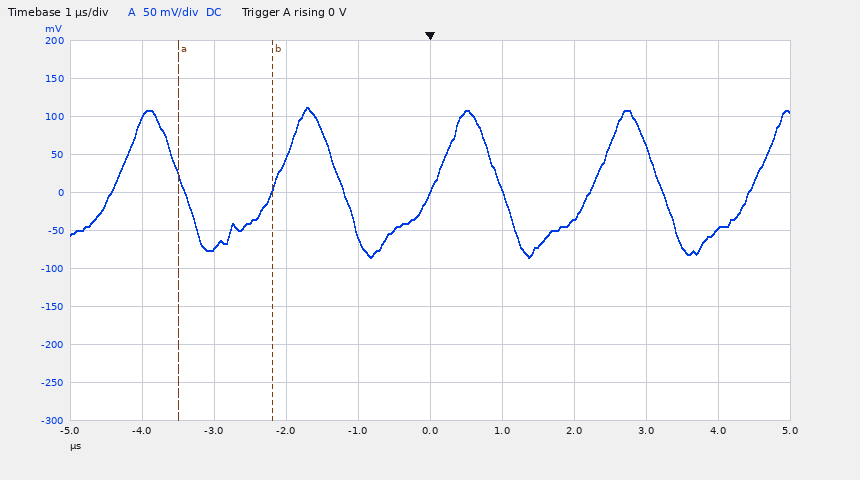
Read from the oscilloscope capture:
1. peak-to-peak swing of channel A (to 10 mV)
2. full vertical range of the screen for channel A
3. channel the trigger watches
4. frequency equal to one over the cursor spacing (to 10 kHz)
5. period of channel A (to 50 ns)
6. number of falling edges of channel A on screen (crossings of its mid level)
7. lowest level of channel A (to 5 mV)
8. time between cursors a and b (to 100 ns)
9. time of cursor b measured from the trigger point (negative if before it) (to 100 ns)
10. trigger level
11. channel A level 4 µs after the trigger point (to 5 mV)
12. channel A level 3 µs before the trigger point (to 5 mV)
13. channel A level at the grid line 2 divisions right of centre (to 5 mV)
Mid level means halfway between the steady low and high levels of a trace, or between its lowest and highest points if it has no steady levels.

200 mV
500 mV
channel A
770 kHz
2.20 µs
4
-85 mV
1.3 µs
-2.2 µs
0 V
-50 mV
-75 mV
-35 mV
